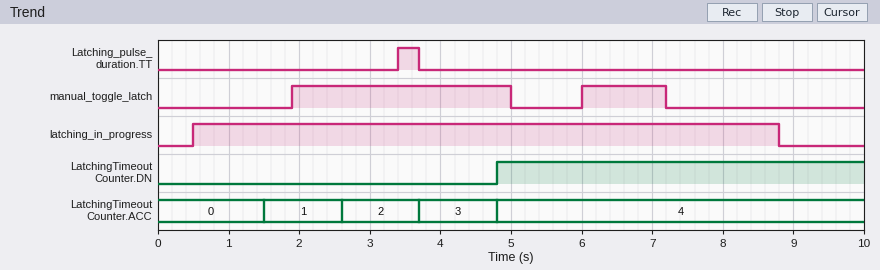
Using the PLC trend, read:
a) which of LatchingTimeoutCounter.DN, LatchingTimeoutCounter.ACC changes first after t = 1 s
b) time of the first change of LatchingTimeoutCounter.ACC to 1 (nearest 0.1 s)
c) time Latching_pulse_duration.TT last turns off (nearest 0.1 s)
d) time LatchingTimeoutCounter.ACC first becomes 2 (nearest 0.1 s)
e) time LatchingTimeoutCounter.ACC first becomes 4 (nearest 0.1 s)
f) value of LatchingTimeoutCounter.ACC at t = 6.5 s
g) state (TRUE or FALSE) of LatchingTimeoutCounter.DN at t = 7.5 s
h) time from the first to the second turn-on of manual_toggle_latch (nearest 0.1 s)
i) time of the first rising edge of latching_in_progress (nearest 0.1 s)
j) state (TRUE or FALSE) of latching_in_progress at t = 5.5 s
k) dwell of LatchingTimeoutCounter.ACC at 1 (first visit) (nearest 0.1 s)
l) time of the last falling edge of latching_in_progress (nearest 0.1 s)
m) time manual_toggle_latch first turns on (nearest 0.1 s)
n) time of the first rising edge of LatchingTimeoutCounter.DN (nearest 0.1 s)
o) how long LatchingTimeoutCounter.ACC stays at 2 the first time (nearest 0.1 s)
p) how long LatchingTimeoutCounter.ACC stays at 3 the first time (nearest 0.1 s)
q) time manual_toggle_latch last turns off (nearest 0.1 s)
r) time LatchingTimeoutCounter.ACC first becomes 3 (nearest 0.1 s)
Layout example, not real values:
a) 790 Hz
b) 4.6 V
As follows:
a) LatchingTimeoutCounter.ACC
b) 1.5 s
c) 3.7 s
d) 2.6 s
e) 4.8 s
f) 4
g) TRUE
h) 4.1 s
i) 0.5 s
j) TRUE
k) 1.1 s
l) 8.8 s
m) 1.9 s
n) 4.8 s
o) 1.1 s
p) 1.1 s
q) 7.2 s
r) 3.7 s
